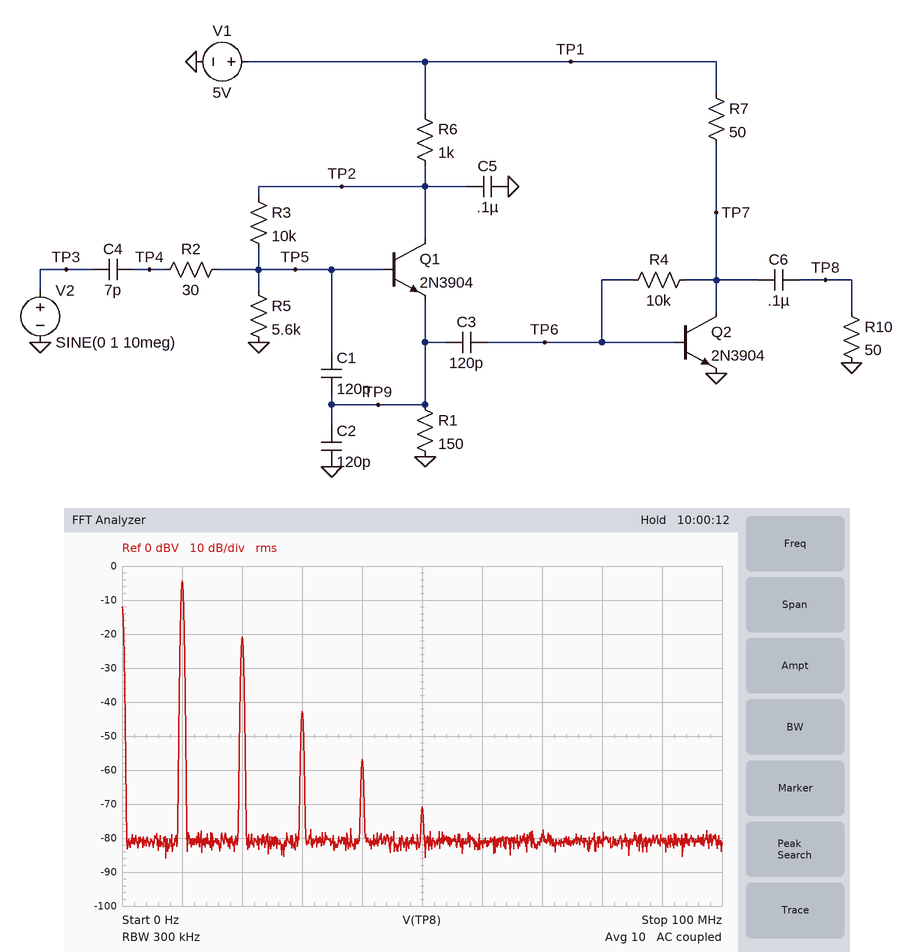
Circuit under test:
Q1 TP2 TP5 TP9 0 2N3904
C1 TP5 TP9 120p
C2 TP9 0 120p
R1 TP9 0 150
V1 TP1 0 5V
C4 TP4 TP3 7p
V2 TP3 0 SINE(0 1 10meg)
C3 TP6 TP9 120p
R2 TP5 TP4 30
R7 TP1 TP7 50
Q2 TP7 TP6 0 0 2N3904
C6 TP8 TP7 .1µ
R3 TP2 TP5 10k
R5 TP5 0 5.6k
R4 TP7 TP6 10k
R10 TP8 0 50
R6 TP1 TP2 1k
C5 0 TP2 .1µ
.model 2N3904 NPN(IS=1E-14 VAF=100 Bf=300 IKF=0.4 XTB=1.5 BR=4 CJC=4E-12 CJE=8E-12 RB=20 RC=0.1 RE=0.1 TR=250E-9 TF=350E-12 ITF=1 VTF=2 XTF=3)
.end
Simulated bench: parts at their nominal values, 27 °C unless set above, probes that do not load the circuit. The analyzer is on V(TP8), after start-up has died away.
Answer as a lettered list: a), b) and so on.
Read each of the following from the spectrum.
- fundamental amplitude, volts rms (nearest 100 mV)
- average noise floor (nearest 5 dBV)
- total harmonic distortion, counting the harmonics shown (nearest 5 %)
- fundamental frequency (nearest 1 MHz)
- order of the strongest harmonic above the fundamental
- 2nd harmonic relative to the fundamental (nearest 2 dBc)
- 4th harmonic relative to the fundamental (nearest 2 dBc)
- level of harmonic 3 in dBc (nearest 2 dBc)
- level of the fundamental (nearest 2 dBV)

a) 600 mV
b) -80 dBV
c) 15 %
d) 10 MHz
e) 2
f) -16 dBc
g) -52 dBc
h) -38 dBc
i) -4 dBV
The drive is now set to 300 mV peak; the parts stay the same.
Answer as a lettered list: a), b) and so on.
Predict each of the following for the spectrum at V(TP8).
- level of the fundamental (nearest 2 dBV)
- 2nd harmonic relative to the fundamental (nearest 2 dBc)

a) -14 dBV
b) -26 dBc
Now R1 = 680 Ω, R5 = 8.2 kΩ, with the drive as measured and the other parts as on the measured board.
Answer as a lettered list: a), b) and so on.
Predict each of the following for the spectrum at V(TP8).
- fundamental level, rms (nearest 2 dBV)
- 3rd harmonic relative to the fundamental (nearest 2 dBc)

a) -6 dBV
b) -34 dBc
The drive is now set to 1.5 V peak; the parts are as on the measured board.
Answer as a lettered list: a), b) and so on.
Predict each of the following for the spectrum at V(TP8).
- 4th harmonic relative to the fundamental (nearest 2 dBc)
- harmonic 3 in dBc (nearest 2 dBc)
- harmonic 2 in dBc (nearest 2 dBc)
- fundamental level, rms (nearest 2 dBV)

a) -46 dBc
b) -32 dBc
c) -14 dBc
d) -2 dBV
